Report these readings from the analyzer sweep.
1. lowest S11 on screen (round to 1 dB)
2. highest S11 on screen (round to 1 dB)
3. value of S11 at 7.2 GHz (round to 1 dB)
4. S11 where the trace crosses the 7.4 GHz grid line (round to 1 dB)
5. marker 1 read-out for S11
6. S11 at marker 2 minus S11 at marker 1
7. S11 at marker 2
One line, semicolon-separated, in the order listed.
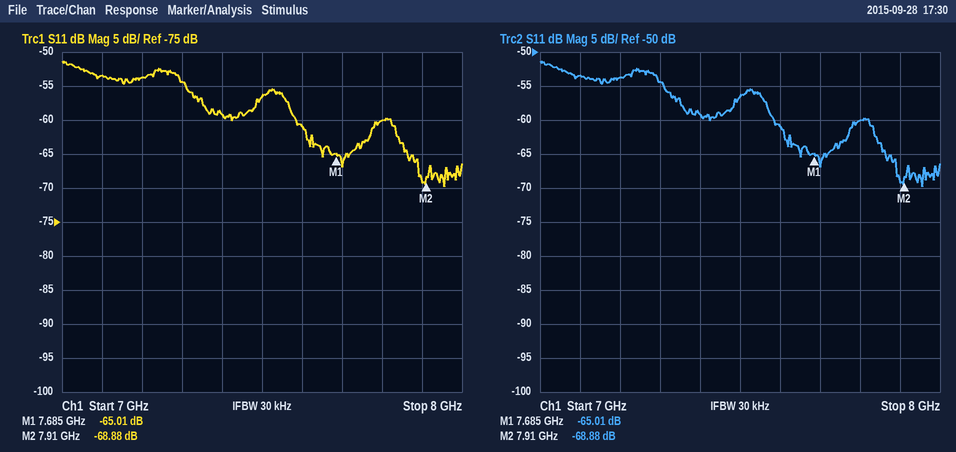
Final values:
-70 dB; -51 dB; -54 dB; -59 dB; -65.01 dB; -3.87 dB; -68.88 dB
